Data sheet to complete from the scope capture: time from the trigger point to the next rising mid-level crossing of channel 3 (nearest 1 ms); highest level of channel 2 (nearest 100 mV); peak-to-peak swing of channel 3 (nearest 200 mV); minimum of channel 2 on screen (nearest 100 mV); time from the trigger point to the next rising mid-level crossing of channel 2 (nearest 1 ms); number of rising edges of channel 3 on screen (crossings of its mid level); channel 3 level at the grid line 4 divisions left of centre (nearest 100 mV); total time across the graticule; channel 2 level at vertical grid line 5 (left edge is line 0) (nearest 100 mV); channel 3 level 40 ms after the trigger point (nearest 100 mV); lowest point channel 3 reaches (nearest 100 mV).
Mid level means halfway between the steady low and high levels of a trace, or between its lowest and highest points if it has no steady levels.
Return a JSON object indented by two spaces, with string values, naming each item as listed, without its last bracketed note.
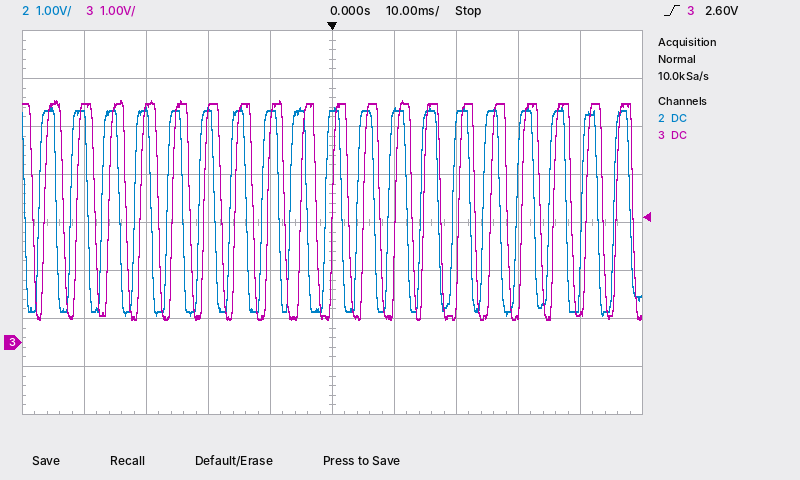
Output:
{
  "time from the trigger point to the next rising mid-level crossing of channel 3": "5 ms",
  "highest level of channel 2": "4.9 V",
  "peak-to-peak swing of channel 3": "4.6 V",
  "minimum of channel 2 on screen": "600 mV",
  "time from the trigger point to the next rising mid-level crossing of channel 2": "4 ms",
  "number of rising edges of channel 3 on screen": "19",
  "channel 3 level at the grid line 4 divisions left of centre": "4.9 V",
  "total time across the graticule": "100 ms",
  "channel 2 level at vertical grid line 5 (left edge is line 0)": "4.8 V",
  "channel 3 level 40 ms after the trigger point": "600 mV",
  "lowest point channel 3 reaches": "500 mV"
}
